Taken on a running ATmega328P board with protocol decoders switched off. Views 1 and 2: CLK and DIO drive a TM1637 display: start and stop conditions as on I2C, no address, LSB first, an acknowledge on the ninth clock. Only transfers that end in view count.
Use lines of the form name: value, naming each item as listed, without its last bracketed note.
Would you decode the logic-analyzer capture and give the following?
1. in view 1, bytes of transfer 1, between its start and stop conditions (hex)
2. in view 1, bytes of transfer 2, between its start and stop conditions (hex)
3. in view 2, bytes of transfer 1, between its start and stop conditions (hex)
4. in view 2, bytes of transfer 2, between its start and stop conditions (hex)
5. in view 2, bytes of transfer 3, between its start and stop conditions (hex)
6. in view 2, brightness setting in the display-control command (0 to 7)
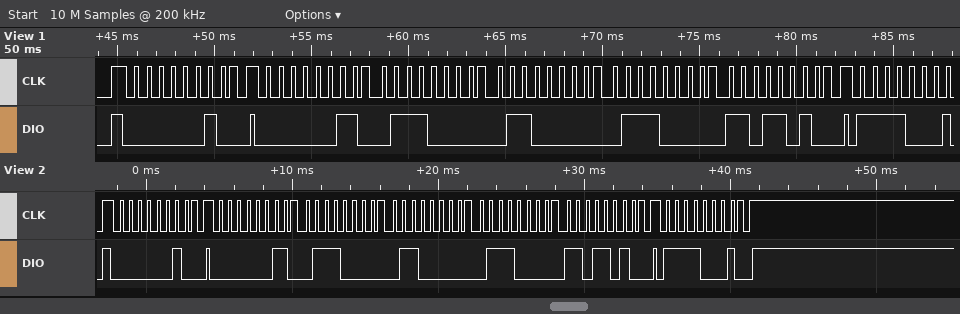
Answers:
in view 1, bytes of transfer 1, between its start and stop conditions: 40
in view 1, bytes of transfer 2, between its start and stop conditions: C0 0E 06 0E 5B
in view 2, bytes of transfer 1, between its start and stop conditions: 40
in view 2, bytes of transfer 2, between its start and stop conditions: C0 0E 06 0E 5B
in view 2, bytes of transfer 3, between its start and stop conditions: 8F
in view 2, brightness setting in the display-control command: 7
